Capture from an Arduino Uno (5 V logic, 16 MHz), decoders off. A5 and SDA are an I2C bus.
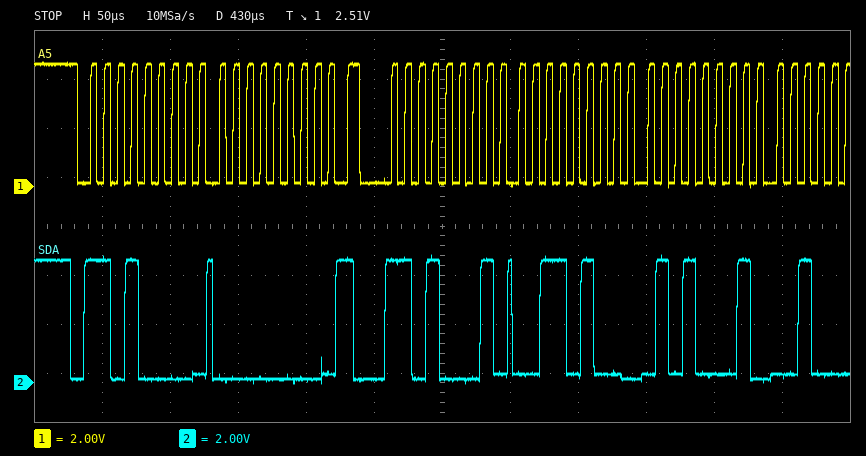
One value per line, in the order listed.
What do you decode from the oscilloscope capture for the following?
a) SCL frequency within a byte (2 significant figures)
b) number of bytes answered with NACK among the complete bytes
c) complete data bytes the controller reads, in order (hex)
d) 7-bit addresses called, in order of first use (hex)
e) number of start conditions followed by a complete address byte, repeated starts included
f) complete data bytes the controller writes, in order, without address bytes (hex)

100 kHz
0
34 51
0x68
2
00
